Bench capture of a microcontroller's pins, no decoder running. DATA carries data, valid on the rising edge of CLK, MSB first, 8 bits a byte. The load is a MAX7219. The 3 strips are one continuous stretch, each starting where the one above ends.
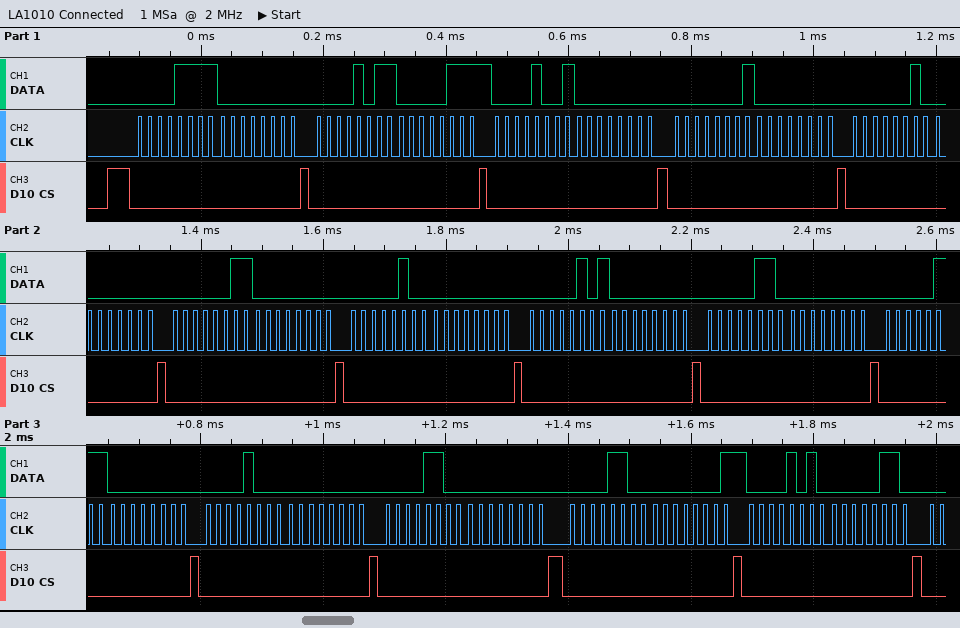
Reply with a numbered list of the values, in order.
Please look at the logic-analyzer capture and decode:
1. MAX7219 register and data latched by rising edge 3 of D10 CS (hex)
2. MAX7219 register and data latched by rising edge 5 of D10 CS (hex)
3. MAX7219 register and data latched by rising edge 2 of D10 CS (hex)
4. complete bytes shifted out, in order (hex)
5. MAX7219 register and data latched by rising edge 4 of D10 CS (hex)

1. register 0xB, data 0x07
2. register 0x1, data 0x00
3. register 0xF, data 0x00
4. 0F 00 0B 07 09 00 01 00 02 00 03 00 04 00 05 00 06 00 07 00 08 00 0C 00 0C 01 0A 06
5. register 0x9, data 0x00
